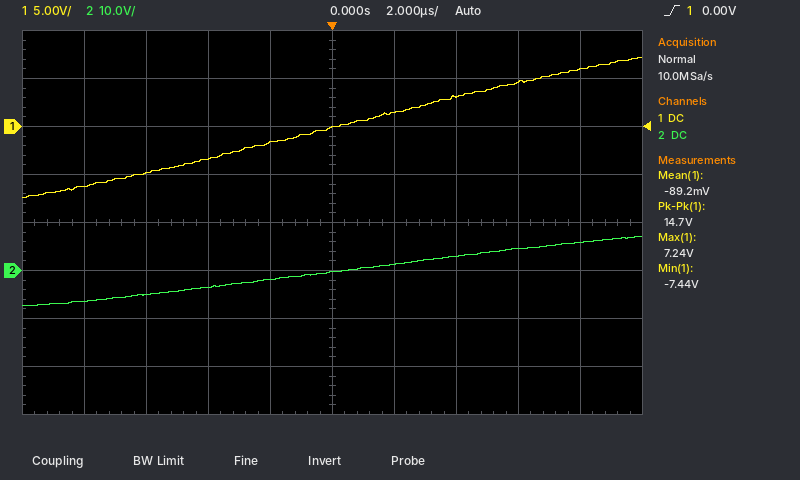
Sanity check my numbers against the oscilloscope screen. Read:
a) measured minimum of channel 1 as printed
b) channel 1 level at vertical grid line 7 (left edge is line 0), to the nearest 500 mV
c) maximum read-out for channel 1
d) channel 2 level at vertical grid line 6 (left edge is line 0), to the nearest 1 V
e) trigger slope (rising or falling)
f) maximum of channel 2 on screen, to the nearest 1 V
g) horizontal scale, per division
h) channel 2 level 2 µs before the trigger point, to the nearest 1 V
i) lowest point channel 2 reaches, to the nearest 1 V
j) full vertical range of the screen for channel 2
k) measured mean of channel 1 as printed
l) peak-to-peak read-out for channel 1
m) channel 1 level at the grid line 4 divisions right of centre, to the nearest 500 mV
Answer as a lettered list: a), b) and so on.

a) -7.44 V
b) 3.0 V
c) 7.24 V
d) 1 V
e) rising
f) 7 V
g) 2 µs
h) -2 V
i) -7 V
j) 80 V
k) -89.2 mV
l) 14.7 V
m) 6.0 V
